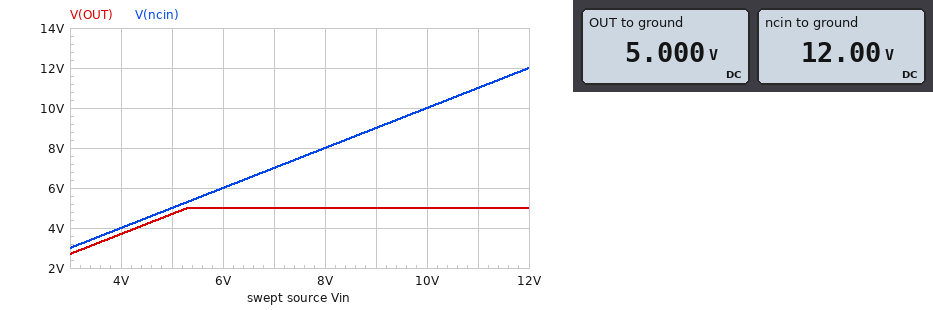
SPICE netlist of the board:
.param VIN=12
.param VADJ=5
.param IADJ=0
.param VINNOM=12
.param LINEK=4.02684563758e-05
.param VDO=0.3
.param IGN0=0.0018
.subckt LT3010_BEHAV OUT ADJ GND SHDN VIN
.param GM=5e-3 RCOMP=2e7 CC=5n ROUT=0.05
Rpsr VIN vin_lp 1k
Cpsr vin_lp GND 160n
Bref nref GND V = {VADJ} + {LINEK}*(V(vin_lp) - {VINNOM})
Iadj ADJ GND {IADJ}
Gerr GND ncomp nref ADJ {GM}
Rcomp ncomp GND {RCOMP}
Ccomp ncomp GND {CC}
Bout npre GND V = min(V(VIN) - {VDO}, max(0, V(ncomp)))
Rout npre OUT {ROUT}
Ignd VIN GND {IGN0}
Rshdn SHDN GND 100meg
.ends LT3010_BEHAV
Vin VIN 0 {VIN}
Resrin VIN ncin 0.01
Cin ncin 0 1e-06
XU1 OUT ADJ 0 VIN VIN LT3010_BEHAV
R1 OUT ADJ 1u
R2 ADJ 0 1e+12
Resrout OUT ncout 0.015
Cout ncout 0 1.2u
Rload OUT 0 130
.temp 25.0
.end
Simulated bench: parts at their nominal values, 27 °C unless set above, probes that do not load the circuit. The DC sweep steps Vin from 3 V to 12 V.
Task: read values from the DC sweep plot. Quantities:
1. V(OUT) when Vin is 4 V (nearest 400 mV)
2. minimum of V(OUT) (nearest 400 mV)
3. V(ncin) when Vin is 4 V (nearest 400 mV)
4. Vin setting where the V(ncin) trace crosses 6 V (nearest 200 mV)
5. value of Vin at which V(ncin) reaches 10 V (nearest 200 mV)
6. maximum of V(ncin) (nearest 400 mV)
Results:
3.6 V
2.8 V
4.0 V
6.0 V
10.0 V
12.0 V
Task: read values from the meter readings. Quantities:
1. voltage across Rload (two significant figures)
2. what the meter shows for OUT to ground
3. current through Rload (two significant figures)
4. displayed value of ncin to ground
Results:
5.0 V
5.000 V
38 mA
12.00 V
